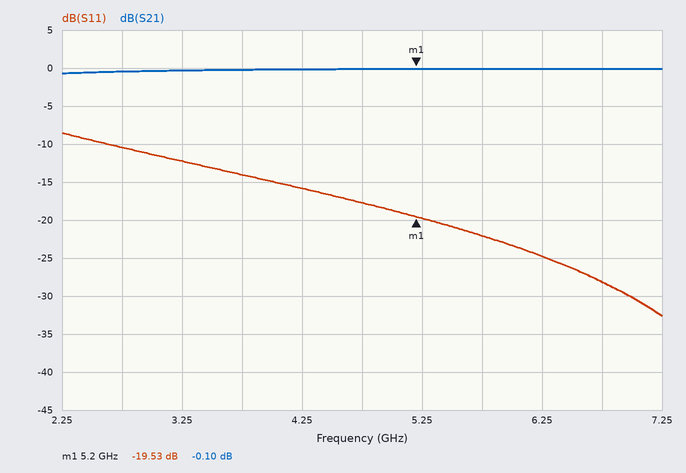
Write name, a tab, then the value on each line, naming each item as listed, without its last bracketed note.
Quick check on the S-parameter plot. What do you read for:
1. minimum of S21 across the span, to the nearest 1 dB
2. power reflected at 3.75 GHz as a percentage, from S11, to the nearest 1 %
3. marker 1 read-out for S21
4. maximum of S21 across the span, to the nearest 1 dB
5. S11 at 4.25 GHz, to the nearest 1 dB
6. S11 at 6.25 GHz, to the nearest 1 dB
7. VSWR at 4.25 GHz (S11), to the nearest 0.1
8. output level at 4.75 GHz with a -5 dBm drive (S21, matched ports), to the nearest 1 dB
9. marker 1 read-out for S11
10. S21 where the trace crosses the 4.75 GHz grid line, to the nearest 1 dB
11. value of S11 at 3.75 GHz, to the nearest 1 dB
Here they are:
minimum of S21 across the span, to the nearest 1 dB	-1 dB
power reflected at 3.75 GHz as a percentage, from S11, to the nearest 1 %	4 %
marker 1 read-out for S21	-0.10 dB
maximum of S21 across the span, to the nearest 1 dB	0 dB
S11 at 4.25 GHz, to the nearest 1 dB	-16 dB
S11 at 6.25 GHz, to the nearest 1 dB	-25 dB
VSWR at 4.25 GHz (S11), to the nearest 0.1	1.4
output level at 4.75 GHz with a -5 dBm drive (S21, matched ports), to the nearest 1 dB	-5 dBm
marker 1 read-out for S11	-19.53 dB
S21 where the trace crosses the 4.75 GHz grid line, to the nearest 1 dB	0 dB
value of S11 at 3.75 GHz, to the nearest 1 dB	-14 dB
